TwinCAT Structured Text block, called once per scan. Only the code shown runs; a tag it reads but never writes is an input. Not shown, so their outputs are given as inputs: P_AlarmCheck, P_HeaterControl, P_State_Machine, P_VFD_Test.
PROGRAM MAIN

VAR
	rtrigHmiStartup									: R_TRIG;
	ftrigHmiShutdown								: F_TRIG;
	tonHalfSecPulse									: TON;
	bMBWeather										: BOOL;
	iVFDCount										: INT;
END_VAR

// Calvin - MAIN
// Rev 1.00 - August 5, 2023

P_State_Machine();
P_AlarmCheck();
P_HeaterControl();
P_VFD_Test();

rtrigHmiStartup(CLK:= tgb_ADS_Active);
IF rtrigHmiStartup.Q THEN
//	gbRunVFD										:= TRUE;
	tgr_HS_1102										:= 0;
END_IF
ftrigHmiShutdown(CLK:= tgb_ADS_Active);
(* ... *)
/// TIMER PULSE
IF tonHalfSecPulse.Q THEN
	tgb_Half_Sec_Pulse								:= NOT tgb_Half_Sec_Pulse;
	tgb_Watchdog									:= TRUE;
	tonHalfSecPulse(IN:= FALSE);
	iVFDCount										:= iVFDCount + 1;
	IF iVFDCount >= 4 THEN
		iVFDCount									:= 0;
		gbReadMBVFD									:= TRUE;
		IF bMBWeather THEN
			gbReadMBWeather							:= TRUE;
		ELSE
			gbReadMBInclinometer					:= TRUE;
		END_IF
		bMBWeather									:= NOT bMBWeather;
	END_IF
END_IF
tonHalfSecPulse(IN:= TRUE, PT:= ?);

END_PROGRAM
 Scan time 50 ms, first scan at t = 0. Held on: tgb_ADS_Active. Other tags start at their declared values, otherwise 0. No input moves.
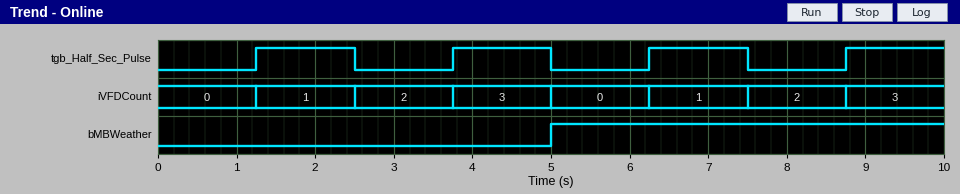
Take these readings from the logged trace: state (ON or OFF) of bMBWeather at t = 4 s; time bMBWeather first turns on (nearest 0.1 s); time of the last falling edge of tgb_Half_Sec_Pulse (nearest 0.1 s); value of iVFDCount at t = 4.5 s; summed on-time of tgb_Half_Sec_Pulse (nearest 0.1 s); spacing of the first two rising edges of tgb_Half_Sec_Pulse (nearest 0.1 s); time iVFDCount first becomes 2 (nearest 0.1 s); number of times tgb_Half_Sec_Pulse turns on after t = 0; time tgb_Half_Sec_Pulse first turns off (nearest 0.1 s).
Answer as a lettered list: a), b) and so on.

a) OFF
b) 5.0 s
c) 7.5 s
d) 3
e) 5.0 s
f) 2.5 s
g) 2.5 s
h) 4
i) 2.5 s
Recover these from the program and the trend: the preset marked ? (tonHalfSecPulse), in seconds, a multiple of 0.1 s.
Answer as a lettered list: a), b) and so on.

a) 1.2 s
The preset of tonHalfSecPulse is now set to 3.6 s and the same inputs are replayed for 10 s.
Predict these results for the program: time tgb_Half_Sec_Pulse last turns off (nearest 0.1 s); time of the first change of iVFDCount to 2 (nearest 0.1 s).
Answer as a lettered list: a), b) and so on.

a) 7.3 s
b) 7.3 s
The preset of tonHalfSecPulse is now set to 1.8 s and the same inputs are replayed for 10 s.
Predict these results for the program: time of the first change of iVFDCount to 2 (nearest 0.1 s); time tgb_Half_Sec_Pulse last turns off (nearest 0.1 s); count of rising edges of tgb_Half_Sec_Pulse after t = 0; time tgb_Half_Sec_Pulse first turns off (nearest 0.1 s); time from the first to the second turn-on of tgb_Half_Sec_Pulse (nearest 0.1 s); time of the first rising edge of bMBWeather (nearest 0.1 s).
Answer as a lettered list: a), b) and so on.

a) 3.7 s
b) 7.4 s
c) 3
d) 3.7 s
e) 3.7 s
f) 7.4 s
